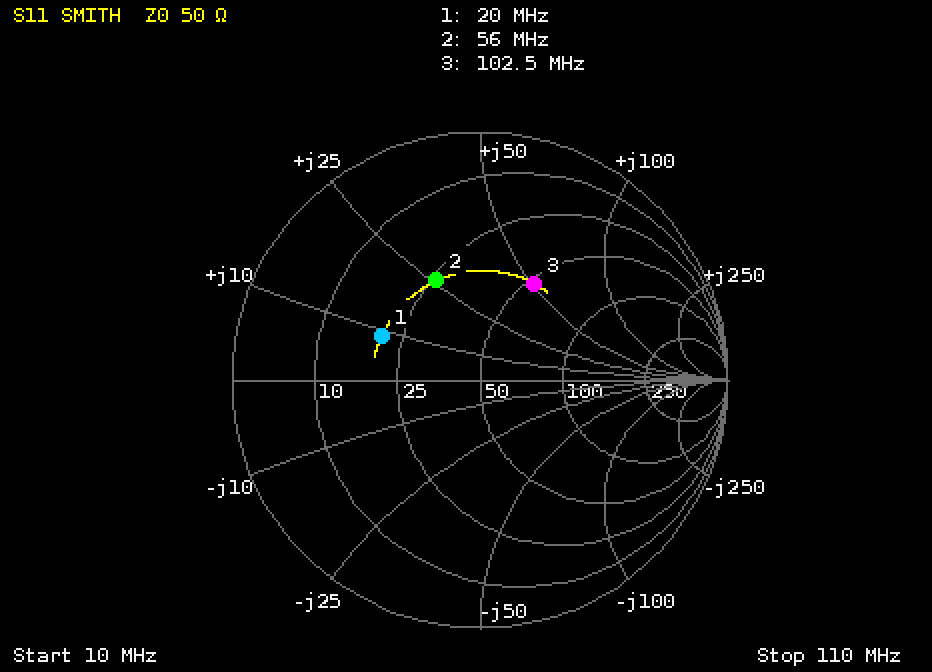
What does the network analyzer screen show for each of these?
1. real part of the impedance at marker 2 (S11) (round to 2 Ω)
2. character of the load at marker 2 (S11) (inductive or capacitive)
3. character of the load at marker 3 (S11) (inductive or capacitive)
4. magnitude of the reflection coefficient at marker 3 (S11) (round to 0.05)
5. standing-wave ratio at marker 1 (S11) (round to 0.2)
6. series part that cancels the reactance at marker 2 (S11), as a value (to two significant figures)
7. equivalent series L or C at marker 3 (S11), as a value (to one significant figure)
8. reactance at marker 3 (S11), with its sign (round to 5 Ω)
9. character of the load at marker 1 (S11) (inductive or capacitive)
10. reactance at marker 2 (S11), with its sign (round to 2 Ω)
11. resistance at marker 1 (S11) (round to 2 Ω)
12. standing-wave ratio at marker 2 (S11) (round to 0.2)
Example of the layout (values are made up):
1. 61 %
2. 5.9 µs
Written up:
1. 26 Ω
2. inductive
3. inductive
4. 0.45
5. 2.6
6. 110 pF
7. 80 nH
8. +50 Ω
9. inductive
10. +26 Ω
11. 20 Ω
12. 2.6
